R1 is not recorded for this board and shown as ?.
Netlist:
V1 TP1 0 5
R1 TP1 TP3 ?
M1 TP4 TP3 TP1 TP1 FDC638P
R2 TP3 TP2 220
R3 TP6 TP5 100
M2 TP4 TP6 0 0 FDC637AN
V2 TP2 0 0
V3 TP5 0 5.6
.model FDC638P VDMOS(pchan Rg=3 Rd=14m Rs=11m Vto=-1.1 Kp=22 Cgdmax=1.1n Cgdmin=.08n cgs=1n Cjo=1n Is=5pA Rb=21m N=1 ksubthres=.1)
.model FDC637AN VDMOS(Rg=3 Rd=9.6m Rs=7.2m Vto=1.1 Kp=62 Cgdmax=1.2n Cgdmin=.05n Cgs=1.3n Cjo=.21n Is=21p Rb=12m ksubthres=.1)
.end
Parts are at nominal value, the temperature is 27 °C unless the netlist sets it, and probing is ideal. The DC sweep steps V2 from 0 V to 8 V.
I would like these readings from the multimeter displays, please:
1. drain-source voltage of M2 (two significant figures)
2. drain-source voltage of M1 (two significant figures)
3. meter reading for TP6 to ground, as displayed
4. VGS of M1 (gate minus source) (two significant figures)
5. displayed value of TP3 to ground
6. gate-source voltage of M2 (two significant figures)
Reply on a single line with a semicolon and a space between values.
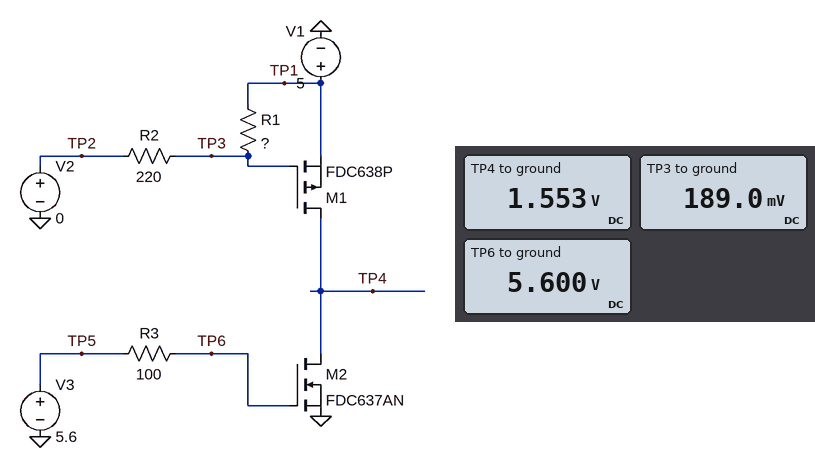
1.6 V; -3.4 V; 5.600 V; -4.8 V; 189.0 mV; 5.6 V
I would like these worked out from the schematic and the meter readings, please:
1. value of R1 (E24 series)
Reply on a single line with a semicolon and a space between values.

5.6 kΩ
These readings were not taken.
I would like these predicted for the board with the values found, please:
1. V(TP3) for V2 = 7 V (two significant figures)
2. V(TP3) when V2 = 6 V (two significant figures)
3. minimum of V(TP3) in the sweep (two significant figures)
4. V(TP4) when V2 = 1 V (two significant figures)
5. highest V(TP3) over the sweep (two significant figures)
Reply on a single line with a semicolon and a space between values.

6.9 V; 6.0 V; 190 mV; 1.1 V; 7.9 V
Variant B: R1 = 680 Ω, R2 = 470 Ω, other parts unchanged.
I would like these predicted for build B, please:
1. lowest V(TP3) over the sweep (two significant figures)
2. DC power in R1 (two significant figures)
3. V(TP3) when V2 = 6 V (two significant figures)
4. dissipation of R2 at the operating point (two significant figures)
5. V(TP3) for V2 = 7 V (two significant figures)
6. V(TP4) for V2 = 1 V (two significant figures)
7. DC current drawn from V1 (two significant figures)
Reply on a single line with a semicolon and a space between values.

2.0 V; 13 mW; 5.6 V; 8.9 mW; 6.2 V; 280 mV; 27 A
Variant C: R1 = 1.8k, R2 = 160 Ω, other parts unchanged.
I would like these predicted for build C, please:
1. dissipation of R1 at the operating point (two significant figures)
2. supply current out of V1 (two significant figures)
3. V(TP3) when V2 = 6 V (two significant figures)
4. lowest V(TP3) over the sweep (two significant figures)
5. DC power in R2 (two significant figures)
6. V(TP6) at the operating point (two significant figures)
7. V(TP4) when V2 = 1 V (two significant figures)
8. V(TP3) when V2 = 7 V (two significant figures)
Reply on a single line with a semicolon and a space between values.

12 mW; 71 A; 5.9 V; 410 mV; 1.0 mW; 5.6 V; 970 mV; 6.8 V
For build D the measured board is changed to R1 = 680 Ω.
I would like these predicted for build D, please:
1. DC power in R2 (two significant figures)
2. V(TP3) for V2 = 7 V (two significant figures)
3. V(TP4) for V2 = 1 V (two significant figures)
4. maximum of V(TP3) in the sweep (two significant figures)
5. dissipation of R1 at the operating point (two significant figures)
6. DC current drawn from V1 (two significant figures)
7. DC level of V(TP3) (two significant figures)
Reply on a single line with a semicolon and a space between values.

6.8 mW; 6.5 V; 590 mV; 7.3 V; 21 mW; 50 A; 1.2 V
